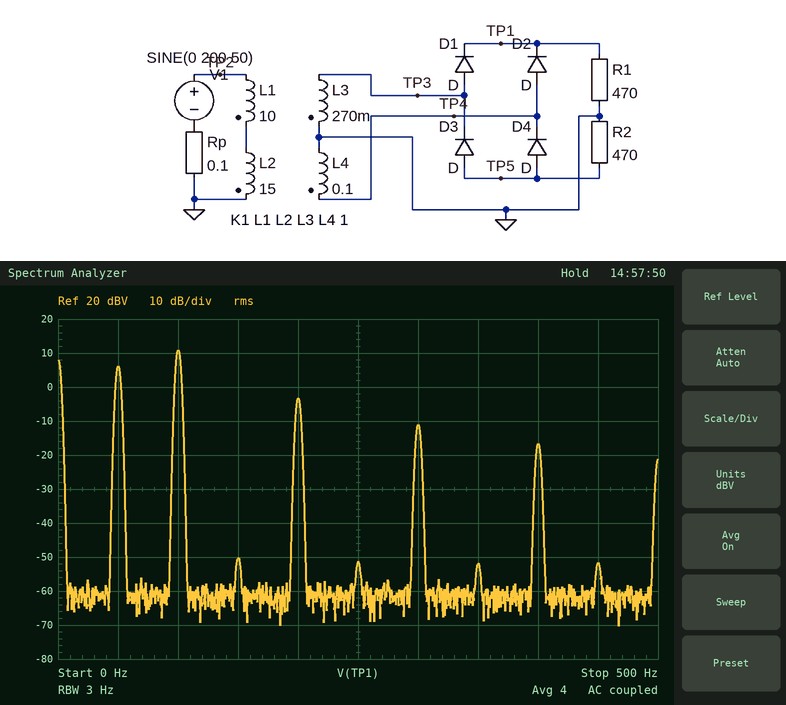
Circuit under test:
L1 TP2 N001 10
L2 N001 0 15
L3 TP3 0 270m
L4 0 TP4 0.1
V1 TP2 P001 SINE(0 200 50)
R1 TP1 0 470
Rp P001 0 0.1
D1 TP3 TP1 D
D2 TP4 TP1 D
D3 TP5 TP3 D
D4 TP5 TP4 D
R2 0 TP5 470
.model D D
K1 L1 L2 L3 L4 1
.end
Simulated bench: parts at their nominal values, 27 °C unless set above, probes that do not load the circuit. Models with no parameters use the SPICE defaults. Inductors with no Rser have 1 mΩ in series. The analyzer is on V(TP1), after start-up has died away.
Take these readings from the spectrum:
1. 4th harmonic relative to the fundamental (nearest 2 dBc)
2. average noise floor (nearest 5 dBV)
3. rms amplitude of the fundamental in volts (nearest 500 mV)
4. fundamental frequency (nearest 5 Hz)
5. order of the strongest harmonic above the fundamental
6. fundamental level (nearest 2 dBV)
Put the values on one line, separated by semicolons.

-10 dBc; -60 dBV; 2.0 V; 50 Hz; 2; 6 dBV
